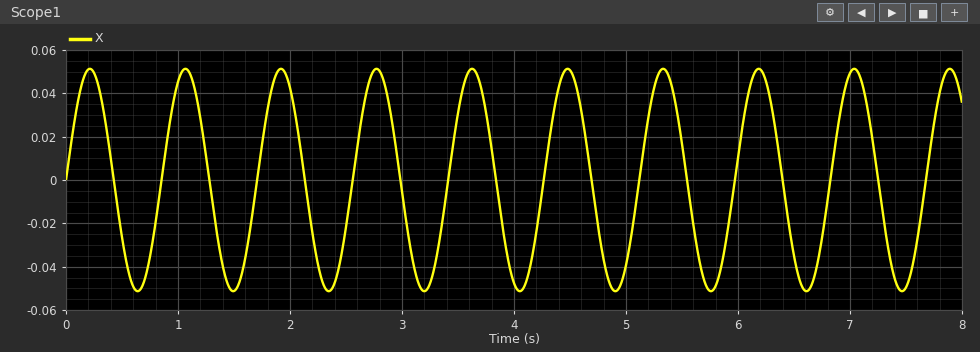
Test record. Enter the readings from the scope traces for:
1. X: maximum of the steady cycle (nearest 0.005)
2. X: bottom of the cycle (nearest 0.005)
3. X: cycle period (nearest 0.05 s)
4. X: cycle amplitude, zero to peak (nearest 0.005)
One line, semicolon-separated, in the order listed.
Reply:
0.050; -0.050; 0.85 s; 0.050
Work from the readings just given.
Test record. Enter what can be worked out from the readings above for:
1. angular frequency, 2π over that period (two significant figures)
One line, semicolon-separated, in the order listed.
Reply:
7.4 rad/s
